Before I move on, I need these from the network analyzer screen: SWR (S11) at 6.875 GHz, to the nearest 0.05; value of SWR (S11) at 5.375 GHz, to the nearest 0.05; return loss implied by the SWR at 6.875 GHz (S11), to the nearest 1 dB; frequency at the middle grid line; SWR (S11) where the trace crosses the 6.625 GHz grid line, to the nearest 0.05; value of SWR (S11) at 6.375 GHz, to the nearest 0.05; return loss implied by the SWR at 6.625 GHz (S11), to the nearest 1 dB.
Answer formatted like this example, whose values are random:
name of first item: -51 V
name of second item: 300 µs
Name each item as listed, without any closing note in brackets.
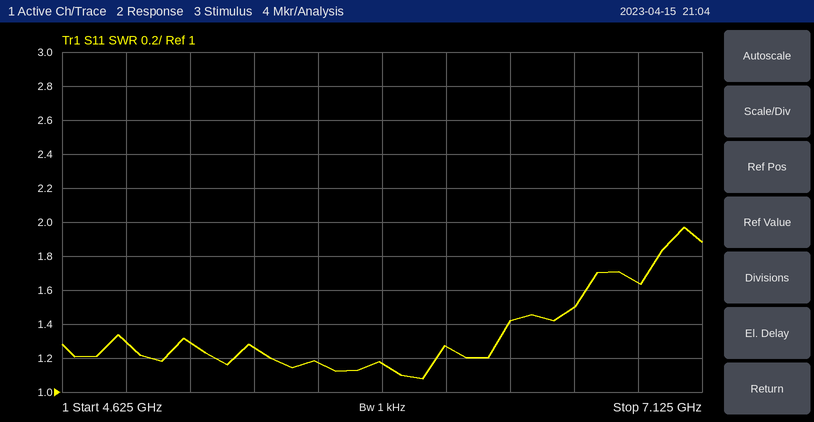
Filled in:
SWR (S11) at 6.875 GHz, to the nearest 0.05: 1.65
value of SWR (S11) at 5.375 GHz, to the nearest 0.05: 1.25
return loss implied by the SWR at 6.875 GHz (S11), to the nearest 1 dB: 12 dB
frequency at the middle grid line: 5.875 GHz
SWR (S11) where the trace crosses the 6.625 GHz grid line, to the nearest 0.05: 1.50
value of SWR (S11) at 6.375 GHz, to the nearest 0.05: 1.40
return loss implied by the SWR at 6.625 GHz (S11), to the nearest 1 dB: 14 dB
